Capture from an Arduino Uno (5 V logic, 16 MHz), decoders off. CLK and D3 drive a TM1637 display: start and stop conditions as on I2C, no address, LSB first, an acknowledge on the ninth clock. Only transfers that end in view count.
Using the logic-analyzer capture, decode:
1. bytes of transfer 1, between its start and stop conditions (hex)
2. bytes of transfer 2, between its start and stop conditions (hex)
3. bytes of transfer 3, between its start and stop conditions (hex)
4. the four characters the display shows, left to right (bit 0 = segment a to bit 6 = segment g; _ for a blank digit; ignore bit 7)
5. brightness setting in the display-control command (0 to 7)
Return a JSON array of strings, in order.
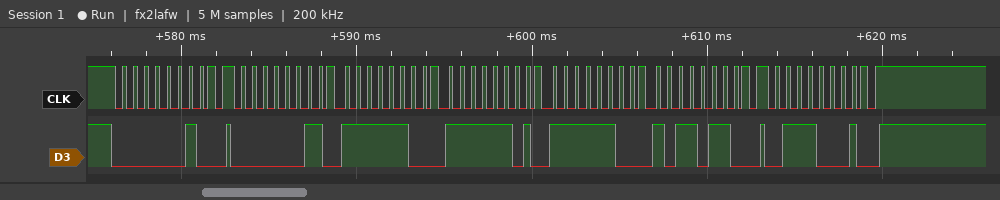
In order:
["40", "C0 3F BF 3F 6D", "8E", "0005", "6"]
